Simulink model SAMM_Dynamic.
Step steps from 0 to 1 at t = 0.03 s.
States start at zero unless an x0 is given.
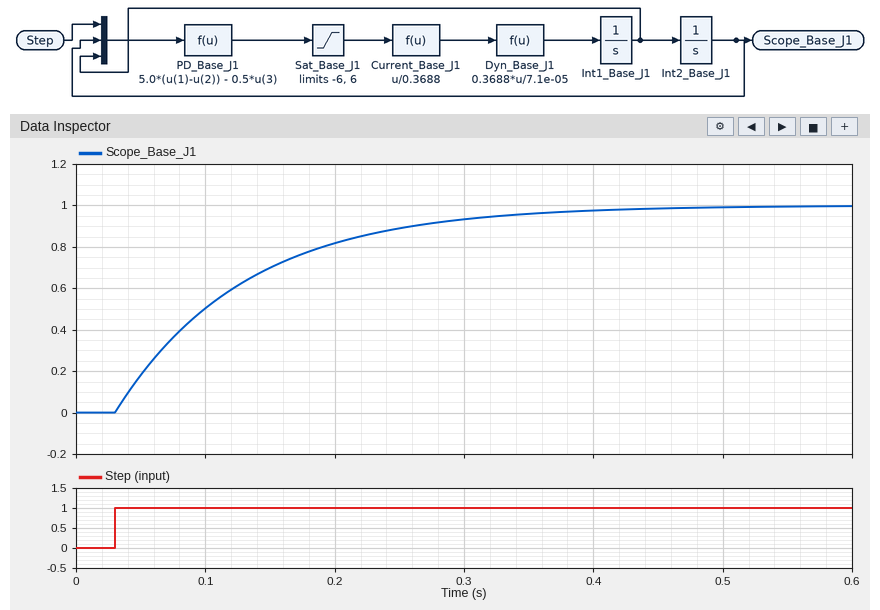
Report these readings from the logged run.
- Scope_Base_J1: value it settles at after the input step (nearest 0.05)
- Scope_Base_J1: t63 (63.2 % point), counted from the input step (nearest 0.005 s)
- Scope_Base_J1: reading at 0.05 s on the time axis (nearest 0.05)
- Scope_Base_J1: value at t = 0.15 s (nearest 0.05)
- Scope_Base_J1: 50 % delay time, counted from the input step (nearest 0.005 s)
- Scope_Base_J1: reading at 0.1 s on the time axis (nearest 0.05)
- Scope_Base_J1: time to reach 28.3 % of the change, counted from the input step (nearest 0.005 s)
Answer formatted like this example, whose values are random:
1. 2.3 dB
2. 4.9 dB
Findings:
1. 1.00
2. 0.100 s
3. 0.20
4. 0.70
5. 0.070 s
6. 0.50
7. 0.035 s
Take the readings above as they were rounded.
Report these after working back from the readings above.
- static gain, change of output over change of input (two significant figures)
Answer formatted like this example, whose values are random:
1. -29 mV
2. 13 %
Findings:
1. 1.0
